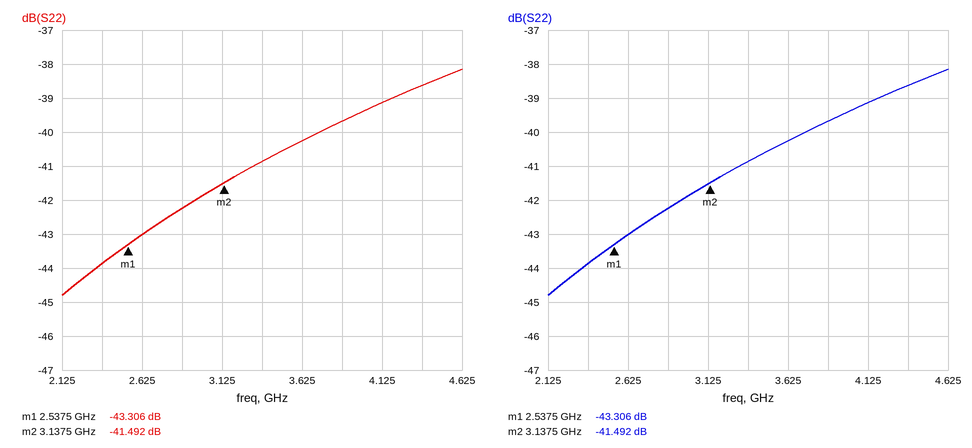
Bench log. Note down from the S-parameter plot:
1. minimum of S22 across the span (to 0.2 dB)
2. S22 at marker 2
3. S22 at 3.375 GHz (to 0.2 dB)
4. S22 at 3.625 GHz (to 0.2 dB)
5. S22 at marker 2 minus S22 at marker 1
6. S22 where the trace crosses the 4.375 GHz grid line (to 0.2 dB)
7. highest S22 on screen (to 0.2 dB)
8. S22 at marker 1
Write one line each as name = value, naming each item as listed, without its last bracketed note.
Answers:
minimum of S22 across the span = -44.8 dB
S22 at marker 2 = -41.492 dB
S22 at 3.375 GHz = -40.8 dB
S22 at 3.625 GHz = -40.2 dB
S22 at marker 2 minus S22 at marker 1 = 1.814 dB
S22 where the trace crosses the 4.375 GHz grid line = -38.6 dB
highest S22 on screen = -38.2 dB
S22 at marker 1 = -43.306 dB
